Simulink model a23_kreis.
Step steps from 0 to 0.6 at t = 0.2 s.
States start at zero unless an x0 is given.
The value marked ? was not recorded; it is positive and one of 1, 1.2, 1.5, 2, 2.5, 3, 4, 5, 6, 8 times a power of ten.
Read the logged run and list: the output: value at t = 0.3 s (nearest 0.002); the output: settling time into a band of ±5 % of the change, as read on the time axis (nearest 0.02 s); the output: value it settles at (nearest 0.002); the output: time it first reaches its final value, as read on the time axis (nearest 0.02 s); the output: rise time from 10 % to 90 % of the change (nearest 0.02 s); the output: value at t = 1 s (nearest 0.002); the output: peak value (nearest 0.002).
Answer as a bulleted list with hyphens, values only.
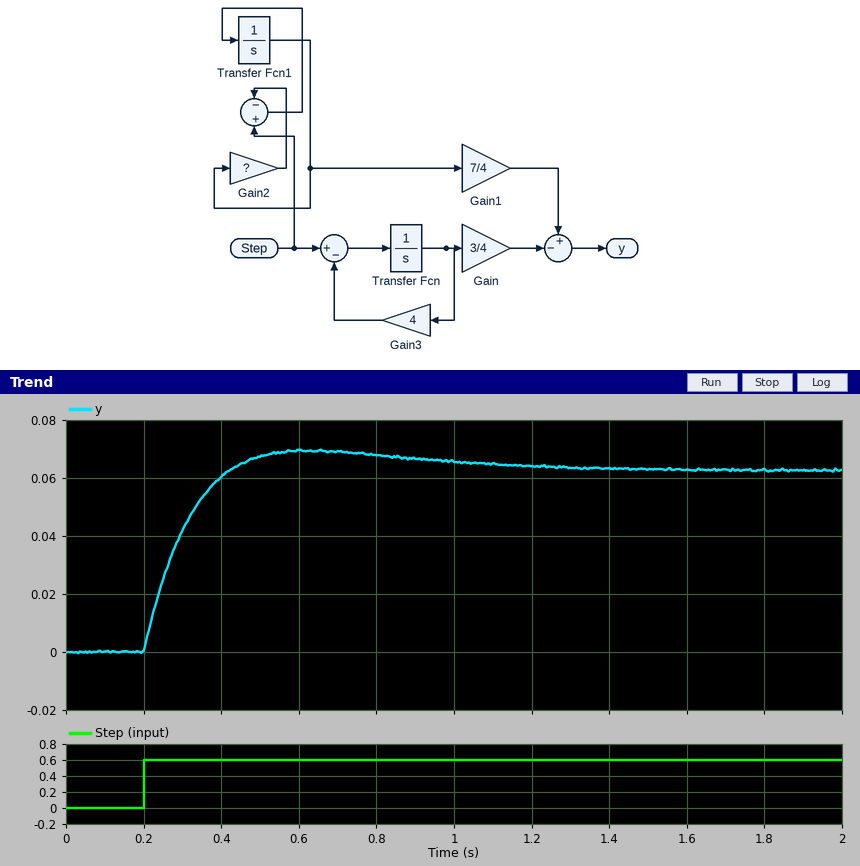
- 0.042
- 1.00 s
- 0.062
- 0.42 s
- 0.16 s
- 0.066
- 0.070
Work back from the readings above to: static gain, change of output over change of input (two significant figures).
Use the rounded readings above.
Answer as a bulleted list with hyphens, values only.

- 0.10
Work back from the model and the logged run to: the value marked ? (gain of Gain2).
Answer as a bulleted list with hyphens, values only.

- 6
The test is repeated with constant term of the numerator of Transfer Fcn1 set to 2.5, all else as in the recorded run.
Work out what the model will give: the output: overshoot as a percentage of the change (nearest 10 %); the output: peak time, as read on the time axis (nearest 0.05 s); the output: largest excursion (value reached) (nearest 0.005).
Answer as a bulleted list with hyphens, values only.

- 70 %
- 0.35 s
- 0.105
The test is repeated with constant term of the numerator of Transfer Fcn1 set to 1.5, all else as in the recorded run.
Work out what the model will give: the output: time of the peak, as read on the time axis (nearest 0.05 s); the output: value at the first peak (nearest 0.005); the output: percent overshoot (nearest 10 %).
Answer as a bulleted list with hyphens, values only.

- 0.45 s
- 0.085
- 40 %
